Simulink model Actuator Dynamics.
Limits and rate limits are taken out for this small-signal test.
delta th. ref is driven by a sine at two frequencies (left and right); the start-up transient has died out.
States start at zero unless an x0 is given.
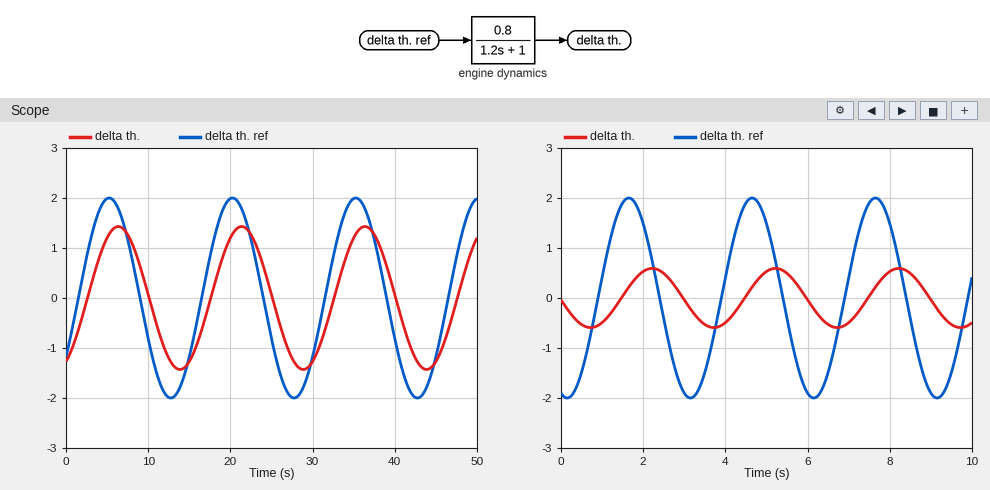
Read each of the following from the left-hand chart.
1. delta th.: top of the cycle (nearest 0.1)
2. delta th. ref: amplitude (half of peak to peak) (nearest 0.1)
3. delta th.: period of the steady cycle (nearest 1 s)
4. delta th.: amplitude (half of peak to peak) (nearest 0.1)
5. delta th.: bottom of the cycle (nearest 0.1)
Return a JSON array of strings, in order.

["1.4", "2.0", "15 s", "1.4", "-1.4"]
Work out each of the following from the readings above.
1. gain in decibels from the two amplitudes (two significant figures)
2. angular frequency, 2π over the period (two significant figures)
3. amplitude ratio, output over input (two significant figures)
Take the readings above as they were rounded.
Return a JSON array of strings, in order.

["-3.1 dB", "0.42 rad/s", "0.70"]
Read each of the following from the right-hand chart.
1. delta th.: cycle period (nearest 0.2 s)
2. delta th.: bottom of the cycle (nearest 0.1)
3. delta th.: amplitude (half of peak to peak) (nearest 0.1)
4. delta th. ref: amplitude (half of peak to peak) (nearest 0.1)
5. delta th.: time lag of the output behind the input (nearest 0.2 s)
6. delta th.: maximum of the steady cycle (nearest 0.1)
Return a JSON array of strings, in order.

["3.0 s", "-0.6", "0.6", "2.0", "0.6 s", "0.6"]
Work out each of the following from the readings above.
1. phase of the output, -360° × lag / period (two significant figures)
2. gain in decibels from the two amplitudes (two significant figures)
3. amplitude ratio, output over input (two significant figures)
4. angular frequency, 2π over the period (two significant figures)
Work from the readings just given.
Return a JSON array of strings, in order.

["-72°", "-10 dB", "0.30", "2.1 rad/s"]
